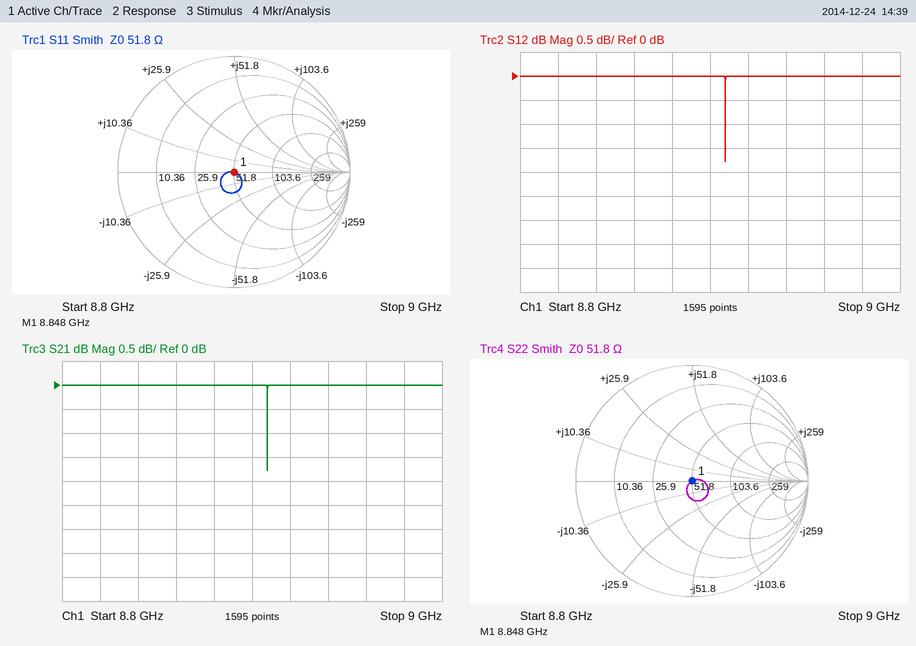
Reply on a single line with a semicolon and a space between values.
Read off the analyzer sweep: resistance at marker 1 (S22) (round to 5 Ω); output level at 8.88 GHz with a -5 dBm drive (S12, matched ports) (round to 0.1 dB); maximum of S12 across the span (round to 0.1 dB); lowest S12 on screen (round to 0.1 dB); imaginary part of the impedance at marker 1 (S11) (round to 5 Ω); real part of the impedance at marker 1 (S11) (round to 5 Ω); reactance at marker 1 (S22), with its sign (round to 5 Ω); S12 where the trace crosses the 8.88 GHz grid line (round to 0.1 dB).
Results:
50 Ω; -5.0 dBm; 0.0 dB; -1.8 dB; 0 Ω; 50 Ω; 0 Ω; 0.0 dB
